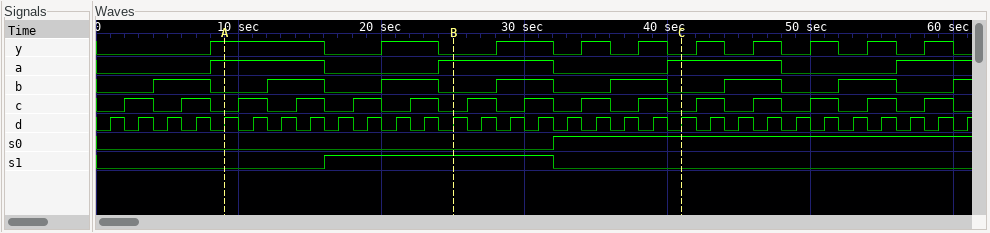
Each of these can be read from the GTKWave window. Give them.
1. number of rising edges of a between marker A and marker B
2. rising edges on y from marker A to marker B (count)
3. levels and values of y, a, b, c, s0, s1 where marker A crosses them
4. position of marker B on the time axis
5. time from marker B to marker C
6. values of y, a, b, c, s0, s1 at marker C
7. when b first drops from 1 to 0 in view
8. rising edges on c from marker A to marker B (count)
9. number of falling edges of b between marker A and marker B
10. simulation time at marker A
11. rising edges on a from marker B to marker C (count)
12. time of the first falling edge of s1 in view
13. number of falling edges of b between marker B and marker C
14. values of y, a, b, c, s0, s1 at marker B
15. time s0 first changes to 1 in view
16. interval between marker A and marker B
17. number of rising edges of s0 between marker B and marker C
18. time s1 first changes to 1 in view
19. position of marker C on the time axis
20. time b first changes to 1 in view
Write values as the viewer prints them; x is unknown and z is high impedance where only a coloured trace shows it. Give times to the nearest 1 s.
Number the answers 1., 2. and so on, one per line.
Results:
1. 1
2. 1
3. y=1, a=1, b=0, c=0, s0=0, s1=0
4. 25 s
5. 16 s
6. y=0, a=1, b=0, c=0, s0=1, s1=0
7. 8 s
8. 4
9. 2
10. 9 s
11. 1
12. 32 s
13. 2
14. y=0, a=1, b=0, c=0, s0=0, s1=1
15. 32 s
16. 16 s
17. 1
18. 16 s
19. 41 s
20. 4 s
